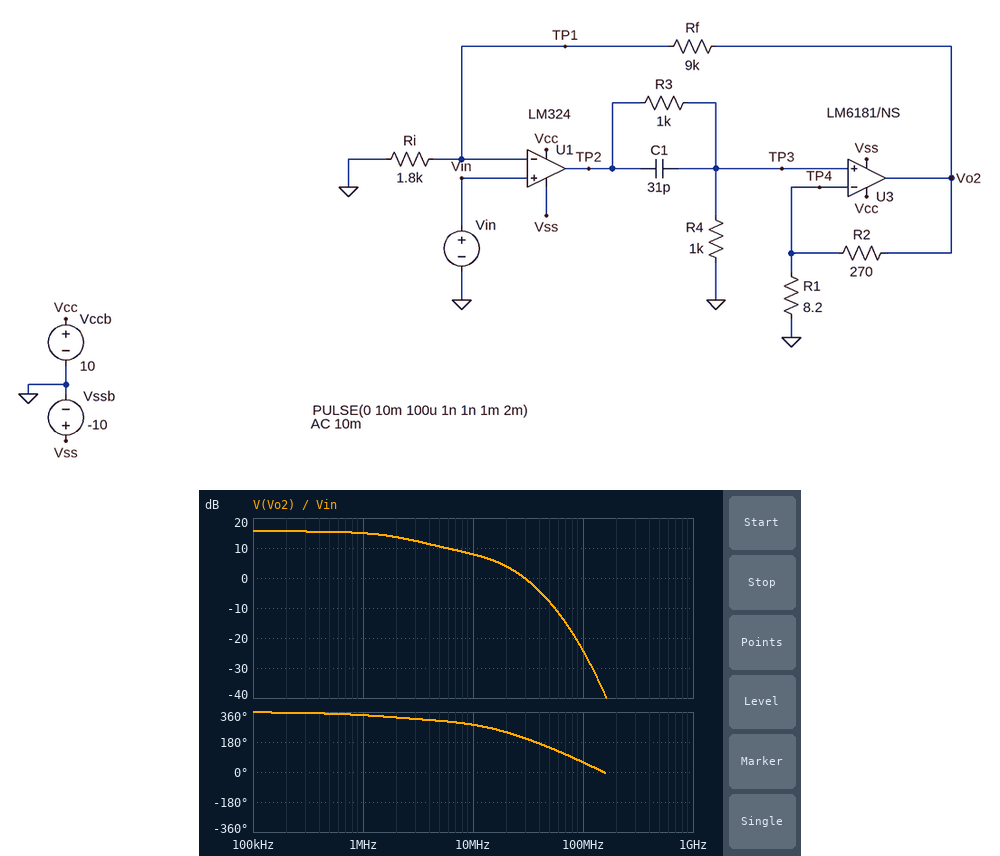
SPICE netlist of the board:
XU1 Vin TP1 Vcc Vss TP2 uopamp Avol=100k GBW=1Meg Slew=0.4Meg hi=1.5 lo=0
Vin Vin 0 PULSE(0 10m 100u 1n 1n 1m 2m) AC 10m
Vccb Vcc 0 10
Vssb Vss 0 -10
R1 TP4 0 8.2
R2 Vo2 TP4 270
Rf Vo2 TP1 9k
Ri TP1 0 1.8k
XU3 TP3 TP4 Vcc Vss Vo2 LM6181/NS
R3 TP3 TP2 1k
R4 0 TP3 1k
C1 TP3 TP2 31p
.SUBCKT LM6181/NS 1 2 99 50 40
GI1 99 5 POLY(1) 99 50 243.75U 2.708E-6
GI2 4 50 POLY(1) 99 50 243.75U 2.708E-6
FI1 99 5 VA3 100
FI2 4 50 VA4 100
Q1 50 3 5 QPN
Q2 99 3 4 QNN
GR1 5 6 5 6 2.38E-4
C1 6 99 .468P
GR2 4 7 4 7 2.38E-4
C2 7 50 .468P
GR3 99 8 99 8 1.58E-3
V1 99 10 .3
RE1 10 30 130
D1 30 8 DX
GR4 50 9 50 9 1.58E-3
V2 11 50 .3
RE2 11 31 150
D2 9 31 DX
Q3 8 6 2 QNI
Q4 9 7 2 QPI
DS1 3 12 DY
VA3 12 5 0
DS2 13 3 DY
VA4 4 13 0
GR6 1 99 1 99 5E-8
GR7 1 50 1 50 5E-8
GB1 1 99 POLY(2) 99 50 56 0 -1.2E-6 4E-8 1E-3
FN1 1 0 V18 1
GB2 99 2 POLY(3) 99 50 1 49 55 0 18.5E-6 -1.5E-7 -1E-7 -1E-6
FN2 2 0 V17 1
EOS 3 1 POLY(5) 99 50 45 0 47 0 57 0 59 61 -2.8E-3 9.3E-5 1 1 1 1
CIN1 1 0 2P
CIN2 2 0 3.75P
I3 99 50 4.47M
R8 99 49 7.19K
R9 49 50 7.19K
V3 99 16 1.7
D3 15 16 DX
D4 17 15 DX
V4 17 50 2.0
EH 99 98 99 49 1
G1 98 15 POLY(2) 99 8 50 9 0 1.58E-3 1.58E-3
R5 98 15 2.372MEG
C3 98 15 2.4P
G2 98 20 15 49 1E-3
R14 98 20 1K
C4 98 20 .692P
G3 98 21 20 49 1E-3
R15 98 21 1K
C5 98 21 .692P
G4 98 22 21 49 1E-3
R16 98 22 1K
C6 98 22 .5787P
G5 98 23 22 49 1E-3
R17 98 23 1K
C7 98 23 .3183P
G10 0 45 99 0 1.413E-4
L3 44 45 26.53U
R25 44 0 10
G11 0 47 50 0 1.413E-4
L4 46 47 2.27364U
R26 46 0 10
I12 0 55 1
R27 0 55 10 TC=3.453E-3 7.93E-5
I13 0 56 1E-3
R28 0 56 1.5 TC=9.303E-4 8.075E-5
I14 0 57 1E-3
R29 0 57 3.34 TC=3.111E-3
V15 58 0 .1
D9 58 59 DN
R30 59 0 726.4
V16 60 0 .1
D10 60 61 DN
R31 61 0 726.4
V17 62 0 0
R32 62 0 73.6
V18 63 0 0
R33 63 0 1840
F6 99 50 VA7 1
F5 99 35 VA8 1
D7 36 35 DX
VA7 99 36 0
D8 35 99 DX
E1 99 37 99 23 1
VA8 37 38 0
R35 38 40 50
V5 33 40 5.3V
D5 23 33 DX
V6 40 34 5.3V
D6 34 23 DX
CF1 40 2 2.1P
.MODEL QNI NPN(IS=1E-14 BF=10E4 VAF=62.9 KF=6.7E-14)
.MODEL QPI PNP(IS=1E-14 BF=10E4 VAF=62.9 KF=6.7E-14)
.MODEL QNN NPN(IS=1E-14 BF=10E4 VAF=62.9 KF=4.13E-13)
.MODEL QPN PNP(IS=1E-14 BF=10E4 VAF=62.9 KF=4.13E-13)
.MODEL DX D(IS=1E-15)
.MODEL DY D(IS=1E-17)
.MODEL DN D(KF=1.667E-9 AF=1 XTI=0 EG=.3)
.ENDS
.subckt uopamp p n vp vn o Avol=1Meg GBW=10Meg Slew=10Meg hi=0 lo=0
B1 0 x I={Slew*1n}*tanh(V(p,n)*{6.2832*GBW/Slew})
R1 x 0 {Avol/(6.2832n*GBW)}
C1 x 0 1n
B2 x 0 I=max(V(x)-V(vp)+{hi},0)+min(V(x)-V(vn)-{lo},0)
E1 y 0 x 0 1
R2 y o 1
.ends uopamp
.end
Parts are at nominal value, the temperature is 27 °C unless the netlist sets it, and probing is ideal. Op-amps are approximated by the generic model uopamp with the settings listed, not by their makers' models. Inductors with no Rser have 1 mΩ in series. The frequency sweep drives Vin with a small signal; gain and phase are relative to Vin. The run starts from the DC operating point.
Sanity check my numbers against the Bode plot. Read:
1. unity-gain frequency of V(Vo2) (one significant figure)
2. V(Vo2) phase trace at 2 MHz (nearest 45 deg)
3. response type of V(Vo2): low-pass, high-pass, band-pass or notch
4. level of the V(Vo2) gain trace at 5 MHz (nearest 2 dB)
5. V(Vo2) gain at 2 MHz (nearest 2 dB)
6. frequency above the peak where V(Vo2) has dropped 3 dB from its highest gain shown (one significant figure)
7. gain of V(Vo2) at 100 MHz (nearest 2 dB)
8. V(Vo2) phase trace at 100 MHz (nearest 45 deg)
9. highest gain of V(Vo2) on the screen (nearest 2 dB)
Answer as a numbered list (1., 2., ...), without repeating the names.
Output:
1. 30 MHz
2. 315 deg
3. low-pass
4. 10 dB
5. 14 dB
6. 3 MHz
7. -24 dB
8. 45 deg
9. 16 dB
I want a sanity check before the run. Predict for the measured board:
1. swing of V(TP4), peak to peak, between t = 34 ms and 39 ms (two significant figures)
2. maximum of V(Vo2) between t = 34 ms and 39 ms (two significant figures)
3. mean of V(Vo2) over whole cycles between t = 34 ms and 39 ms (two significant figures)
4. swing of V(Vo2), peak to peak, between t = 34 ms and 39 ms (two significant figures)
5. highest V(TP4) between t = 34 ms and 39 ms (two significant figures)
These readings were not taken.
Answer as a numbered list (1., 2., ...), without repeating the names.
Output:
1. 1.8 mV
2. 60 mV
3. 30 mV
4. 60 mV
5. 1.8 mV
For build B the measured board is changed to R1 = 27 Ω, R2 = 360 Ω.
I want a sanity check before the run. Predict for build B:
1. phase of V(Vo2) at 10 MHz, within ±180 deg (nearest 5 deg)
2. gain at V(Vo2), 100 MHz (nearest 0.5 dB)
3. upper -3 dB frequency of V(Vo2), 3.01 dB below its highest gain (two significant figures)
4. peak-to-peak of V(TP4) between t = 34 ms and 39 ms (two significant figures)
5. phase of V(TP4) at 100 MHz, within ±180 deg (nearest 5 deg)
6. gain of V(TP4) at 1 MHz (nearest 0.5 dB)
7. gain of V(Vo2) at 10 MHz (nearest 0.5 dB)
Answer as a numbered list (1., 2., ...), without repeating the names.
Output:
1. -80 deg
2. -24.5 dB
3. 1.1 MHz
4. 4.2 mV
5. 140 deg
6. -10.0 dB
7. 0.5 dB
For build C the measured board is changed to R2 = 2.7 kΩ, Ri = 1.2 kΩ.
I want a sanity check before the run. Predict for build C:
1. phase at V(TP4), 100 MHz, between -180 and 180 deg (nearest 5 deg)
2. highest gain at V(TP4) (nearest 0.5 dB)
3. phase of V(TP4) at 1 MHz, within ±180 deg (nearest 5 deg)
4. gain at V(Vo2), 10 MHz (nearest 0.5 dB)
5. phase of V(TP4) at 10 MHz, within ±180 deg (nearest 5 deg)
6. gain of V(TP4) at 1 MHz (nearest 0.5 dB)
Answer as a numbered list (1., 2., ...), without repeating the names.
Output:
1. -170 deg
2. -21.5 dB
3. 0 deg
4. 27.0 dB
5. -45 deg
6. -31.5 dB
